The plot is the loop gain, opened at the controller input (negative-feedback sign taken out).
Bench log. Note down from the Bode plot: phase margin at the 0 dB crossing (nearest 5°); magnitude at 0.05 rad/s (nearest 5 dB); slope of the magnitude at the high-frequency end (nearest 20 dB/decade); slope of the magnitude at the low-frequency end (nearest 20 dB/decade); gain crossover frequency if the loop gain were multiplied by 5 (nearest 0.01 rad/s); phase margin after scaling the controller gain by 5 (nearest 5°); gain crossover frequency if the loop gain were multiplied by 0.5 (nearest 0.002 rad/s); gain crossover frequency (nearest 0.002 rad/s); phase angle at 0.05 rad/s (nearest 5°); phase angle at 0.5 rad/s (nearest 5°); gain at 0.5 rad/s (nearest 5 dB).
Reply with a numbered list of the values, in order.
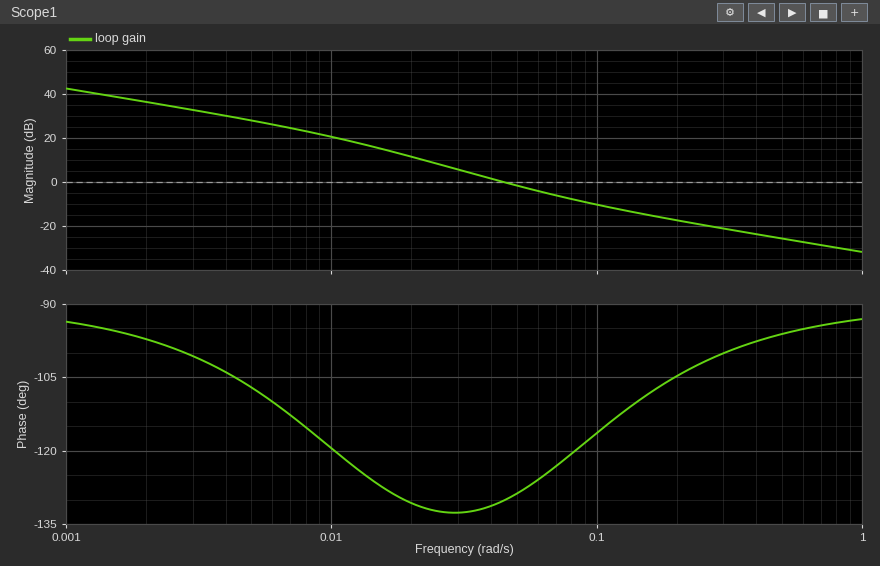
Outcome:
1. 50°
2. 0 dB
3. -20 dB/decade
4. -20 dB/decade
5. 0.14 rad/s
6. 70°
7. 0.030 rad/s
8. 0.044 rad/s
9. -130°
10. -95°
11. -25 dB
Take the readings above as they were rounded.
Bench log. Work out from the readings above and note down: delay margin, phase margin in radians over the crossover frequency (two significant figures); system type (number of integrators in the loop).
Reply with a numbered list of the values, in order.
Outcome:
1. 20 s
2. 1
